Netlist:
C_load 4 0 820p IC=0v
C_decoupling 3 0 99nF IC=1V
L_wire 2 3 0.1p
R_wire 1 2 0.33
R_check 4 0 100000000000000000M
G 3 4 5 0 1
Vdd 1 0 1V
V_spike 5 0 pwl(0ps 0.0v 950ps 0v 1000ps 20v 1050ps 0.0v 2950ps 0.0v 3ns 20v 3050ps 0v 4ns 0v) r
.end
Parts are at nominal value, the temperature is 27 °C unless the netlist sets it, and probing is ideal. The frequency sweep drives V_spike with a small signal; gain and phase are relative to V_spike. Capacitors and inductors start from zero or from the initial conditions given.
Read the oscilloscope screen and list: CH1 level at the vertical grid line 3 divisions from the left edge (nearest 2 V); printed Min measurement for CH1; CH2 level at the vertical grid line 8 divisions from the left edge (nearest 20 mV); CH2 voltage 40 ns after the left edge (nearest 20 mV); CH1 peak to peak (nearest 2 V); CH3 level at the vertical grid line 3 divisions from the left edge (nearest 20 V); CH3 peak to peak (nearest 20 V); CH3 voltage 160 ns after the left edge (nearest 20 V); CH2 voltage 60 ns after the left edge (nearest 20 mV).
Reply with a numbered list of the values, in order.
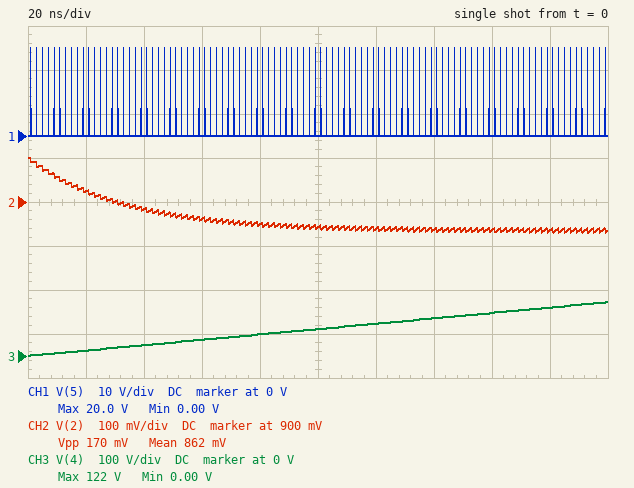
1. 0 V
2. 0.00 V
3. 840 mV
4. 880 mV
5. 20 V
6. 40 V
7. 120 V
8. 100 V
9. 860 mV
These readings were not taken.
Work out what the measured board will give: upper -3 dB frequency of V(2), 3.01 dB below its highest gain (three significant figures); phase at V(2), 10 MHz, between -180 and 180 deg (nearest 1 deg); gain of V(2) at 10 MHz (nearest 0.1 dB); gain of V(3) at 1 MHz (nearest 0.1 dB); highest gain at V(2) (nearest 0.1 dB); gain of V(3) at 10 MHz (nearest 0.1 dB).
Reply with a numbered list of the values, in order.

1. 4.87 MHz
2. 116 deg
3. -16.8 dB
4. -9.8 dB
5. -9.6 dB
6. -16.8 dB
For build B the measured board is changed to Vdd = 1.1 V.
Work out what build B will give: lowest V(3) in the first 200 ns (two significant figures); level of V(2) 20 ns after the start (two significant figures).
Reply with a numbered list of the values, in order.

1. 930 mV
2. 970 mV
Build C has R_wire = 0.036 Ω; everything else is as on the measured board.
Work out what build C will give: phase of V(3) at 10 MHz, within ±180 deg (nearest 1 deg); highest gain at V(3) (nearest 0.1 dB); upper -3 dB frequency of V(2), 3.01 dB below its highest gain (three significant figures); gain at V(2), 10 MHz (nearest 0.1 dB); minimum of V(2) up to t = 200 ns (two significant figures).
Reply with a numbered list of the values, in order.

1. 167 deg
2. -28.9 dB
3. 44.7 MHz
4. -29.1 dB
5. 980 mV
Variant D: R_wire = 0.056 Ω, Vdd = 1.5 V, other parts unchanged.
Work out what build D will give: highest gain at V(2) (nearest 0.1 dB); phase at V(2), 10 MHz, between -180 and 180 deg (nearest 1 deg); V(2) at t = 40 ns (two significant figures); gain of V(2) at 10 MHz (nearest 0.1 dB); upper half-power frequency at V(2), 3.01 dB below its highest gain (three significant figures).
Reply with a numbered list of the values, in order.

1. -25.0 dB
2. 161 deg
3. 1.5 V
4. -25.5 dB
5. 28.7 MHz
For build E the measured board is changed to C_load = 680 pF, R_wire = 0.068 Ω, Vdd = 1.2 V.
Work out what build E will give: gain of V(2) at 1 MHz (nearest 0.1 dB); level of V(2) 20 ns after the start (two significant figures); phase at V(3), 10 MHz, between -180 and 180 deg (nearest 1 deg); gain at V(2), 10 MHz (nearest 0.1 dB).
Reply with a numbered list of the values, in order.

1. -23.4 dB
2. 1.2 V
3. 157 deg
4. -24.1 dB
